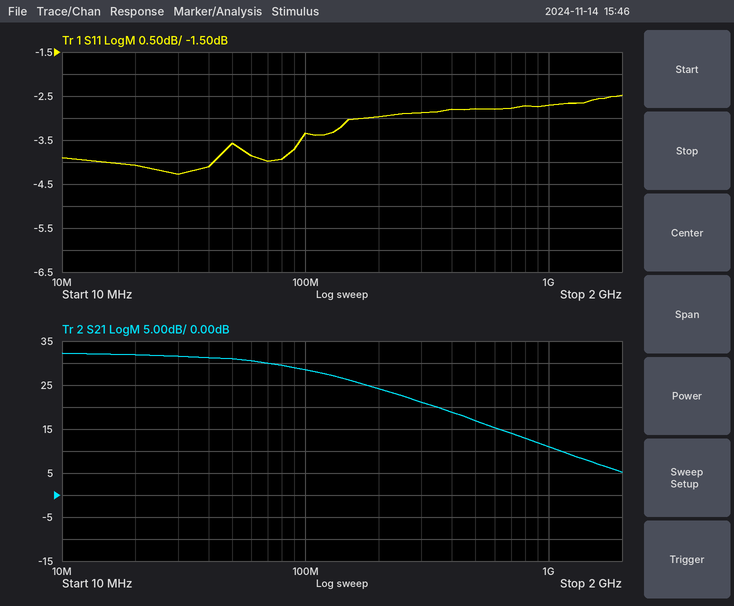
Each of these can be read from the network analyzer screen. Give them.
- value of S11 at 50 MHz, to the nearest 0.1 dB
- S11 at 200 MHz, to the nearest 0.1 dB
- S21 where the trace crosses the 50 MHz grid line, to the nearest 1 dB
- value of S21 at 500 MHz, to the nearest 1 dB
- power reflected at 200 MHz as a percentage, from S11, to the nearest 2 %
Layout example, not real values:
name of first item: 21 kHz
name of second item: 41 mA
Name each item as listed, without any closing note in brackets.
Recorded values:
value of S11 at 50 MHz, to the nearest 0.1 dB: -3.6 dB
S11 at 200 MHz, to the nearest 0.1 dB: -3.0 dB
S21 where the trace crosses the 50 MHz grid line, to the nearest 1 dB: 31 dB
value of S21 at 500 MHz, to the nearest 1 dB: 17 dB
power reflected at 200 MHz as a percentage, from S11, to the nearest 2 %: 50 %
